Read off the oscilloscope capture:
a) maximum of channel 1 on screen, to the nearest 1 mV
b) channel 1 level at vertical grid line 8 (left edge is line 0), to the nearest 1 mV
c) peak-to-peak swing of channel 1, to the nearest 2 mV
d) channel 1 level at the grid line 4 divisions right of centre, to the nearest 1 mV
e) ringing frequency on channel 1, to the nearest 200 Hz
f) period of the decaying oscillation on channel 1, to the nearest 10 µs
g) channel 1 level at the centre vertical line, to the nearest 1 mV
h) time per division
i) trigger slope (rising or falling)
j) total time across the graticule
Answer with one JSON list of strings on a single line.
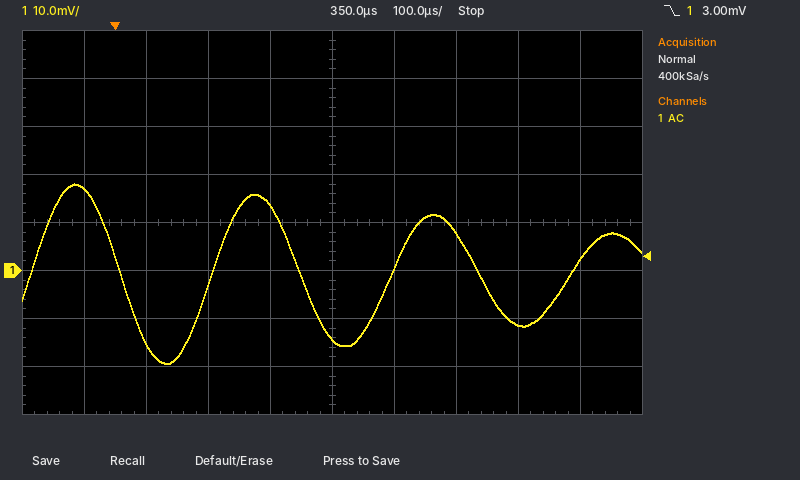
["18 mV", "-11 mV", "38 mV", "2 mV", "3.4 kHz", "290 µs", "-14 mV", "100 µs", "falling", "1 ms"]
